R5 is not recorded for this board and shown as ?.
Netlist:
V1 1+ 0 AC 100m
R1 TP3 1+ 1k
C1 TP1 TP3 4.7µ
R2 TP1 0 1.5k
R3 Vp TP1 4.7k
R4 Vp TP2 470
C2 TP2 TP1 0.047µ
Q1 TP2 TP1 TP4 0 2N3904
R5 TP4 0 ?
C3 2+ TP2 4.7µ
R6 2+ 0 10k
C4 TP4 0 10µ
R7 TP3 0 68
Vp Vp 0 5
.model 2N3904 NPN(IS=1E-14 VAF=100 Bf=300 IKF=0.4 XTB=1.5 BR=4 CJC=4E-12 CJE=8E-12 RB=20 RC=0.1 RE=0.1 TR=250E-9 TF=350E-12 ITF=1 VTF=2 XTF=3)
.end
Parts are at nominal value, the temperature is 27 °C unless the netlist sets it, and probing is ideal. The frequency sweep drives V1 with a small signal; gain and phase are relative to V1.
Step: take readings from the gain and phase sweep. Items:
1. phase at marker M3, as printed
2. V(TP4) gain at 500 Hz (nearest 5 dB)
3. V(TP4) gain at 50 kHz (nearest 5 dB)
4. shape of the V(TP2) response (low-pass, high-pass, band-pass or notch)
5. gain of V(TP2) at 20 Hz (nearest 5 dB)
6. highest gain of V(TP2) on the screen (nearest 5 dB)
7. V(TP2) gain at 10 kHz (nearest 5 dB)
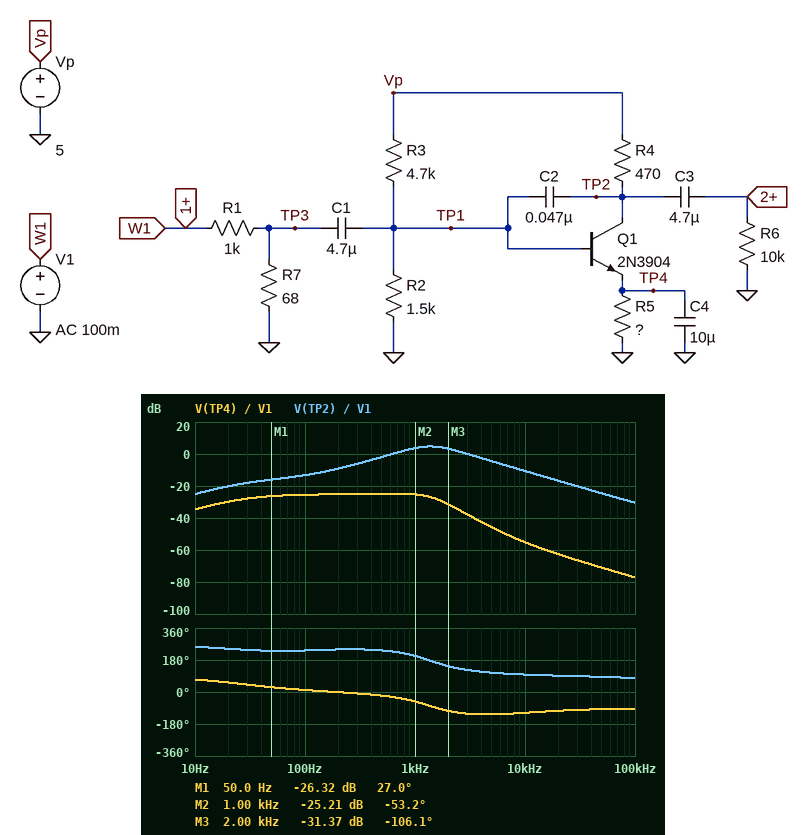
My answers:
-106.1 deg
-25 dB
-70 dB
band-pass
-20 dB
5 dB
-10 dB
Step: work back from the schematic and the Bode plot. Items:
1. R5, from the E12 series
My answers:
150 Ω
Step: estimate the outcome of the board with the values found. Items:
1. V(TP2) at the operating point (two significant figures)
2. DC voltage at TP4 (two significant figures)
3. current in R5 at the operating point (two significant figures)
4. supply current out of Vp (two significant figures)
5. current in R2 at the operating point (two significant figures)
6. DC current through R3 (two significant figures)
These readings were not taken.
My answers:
3.4 V
510 mV
3.4 mA
4.2 mA
800 µA
810 µA
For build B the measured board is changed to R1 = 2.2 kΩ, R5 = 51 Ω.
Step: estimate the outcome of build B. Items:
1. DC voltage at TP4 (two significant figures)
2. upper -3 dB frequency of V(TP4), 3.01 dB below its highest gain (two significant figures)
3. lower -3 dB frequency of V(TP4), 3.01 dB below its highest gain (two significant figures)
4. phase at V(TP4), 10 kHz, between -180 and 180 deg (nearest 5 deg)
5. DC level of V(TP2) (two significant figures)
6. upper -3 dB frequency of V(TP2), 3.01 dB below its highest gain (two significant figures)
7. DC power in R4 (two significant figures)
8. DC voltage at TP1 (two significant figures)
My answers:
460 mV
1.7 kHz
41 Hz
-120 deg
770 mV
2.3 kHz
38 mW
1.2 V
